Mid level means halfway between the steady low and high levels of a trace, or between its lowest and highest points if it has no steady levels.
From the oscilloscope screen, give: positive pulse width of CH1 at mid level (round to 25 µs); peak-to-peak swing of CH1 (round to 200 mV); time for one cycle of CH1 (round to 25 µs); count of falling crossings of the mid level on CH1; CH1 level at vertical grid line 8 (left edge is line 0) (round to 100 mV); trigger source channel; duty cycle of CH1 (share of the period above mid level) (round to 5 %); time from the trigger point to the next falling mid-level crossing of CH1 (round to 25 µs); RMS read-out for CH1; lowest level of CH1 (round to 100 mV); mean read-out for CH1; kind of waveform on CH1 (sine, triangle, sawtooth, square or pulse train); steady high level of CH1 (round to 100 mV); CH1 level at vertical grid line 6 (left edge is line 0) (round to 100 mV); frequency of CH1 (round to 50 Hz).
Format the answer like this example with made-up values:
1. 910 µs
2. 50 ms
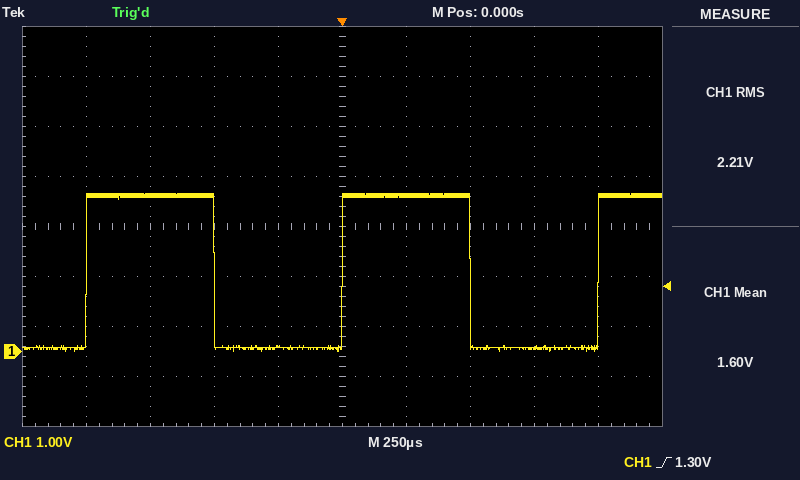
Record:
1. 500 µs
2. 3.2 V
3. 1.000 ms
4. 2
5. 100 mV
6. CH1
7. 50 %
8. 500 µs
9. 2.21 V
10. 0.0 V
11. 1.60 V
12. square
13. 3.1 V
14. 3.1 V
15. 1.00 kHz
